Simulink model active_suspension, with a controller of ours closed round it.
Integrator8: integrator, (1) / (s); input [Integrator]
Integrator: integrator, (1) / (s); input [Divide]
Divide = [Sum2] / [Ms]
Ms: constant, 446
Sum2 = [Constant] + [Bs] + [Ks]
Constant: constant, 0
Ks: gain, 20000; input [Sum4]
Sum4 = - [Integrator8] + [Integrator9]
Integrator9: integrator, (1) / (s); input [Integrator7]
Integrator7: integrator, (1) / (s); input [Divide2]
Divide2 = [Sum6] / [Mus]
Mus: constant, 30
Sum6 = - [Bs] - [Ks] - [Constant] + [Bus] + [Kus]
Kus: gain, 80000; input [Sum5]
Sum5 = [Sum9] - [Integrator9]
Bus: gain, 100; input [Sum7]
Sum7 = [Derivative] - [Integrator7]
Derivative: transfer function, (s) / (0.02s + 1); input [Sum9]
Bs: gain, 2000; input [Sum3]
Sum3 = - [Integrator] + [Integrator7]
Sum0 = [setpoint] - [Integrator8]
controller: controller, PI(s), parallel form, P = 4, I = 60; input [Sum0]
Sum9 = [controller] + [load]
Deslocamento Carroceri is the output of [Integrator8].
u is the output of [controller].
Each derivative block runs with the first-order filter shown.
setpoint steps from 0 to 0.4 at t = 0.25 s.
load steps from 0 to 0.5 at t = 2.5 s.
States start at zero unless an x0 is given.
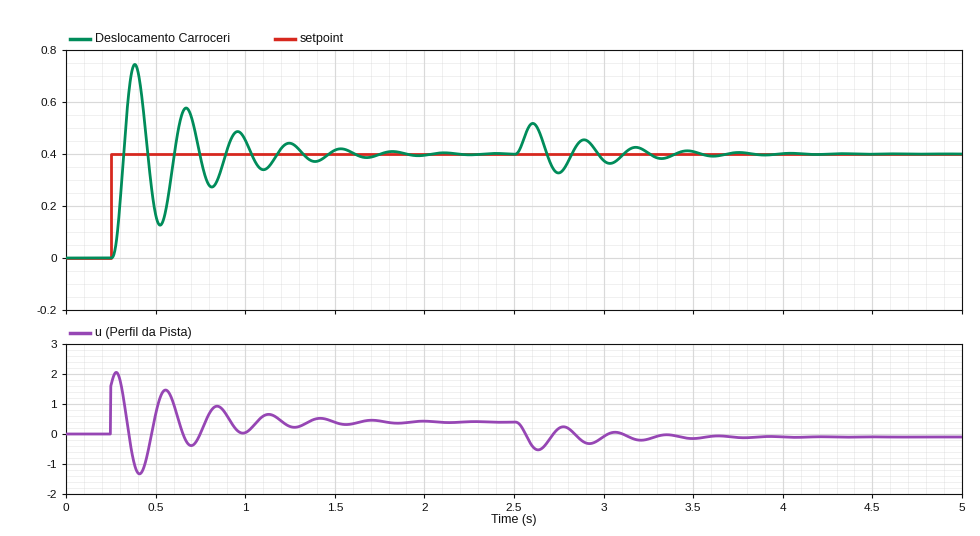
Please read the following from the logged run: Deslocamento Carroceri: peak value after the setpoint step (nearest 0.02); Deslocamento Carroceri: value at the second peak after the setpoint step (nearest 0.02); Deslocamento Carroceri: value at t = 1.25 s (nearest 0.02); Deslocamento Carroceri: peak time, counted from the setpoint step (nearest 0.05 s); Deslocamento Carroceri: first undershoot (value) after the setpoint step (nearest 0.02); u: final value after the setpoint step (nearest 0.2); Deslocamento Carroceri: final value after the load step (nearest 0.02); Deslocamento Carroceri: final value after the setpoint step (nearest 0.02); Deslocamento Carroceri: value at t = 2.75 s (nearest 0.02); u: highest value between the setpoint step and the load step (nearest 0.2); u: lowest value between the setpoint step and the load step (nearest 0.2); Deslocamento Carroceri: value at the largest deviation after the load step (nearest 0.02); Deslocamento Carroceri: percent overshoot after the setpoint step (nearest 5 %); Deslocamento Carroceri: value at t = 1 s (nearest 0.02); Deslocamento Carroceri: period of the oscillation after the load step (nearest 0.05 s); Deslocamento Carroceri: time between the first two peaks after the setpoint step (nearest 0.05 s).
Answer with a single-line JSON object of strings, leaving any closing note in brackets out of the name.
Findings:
{"Deslocamento Carroceri: peak value after the setpoint step": "0.74", "Deslocamento Carroceri: value at the second peak after the setpoint step": "0.58", "Deslocamento Carroceri: value at t = 1.25 s": "0.44", "Deslocamento Carroceri: peak time, counted from the setpoint step": "0.15 s", "Deslocamento Carroceri: first undershoot (value) after the setpoint step": "0.12", "u: final value after the setpoint step": "0.4", "Deslocamento Carroceri: final value after the load step": "0.40", "Deslocamento Carroceri: final value after the setpoint step": "0.40", "Deslocamento Carroceri: value at t = 2.75 s": "0.32", "u: highest value between the setpoint step and the load step": "2.0", "u: lowest value between the setpoint step and the load step": "-1.4", "Deslocamento Carroceri: value at the largest deviation after the load step": "0.52", "Deslocamento Carroceri: percent overshoot after the setpoint step": "85 %", "Deslocamento Carroceri: value at t = 1 s": "0.46", "Deslocamento Carroceri: period of the oscillation after the load step": "0.30 s", "Deslocamento Carroceri: time between the first two peaks after the setpoint step": "0.30 s"}
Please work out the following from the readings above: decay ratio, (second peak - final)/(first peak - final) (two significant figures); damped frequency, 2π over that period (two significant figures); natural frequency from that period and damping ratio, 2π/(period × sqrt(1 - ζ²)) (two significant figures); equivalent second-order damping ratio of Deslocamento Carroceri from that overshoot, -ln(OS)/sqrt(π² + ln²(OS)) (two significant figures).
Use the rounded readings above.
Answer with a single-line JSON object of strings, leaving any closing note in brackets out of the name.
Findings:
{"decay ratio, (second peak - final)/(first peak - final)": "0.53", "damped frequency, 2π over that period": "21 rad/s", "natural frequency from that period and damping ratio, 2π/(period × sqrt(1 - ζ²))": "21 rad/s", "equivalent second-order damping ratio of Deslocamento Carroceri from that overshoot, -ln(OS)/sqrt(π² + ln²(OS))": "0.052"}
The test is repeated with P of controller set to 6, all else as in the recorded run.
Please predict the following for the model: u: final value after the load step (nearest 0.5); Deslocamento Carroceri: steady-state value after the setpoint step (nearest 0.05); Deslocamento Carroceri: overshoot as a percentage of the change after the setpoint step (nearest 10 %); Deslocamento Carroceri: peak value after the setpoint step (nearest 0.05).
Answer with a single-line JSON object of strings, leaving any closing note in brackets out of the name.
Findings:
{"u: final value after the load step": "0.0", "Deslocamento Carroceri: steady-state value after the setpoint step": "0.40", "Deslocamento Carroceri: overshoot as a percentage of the change after the setpoint step": "80 %", "Deslocamento Carroceri: peak value after the setpoint step": "0.70"}
